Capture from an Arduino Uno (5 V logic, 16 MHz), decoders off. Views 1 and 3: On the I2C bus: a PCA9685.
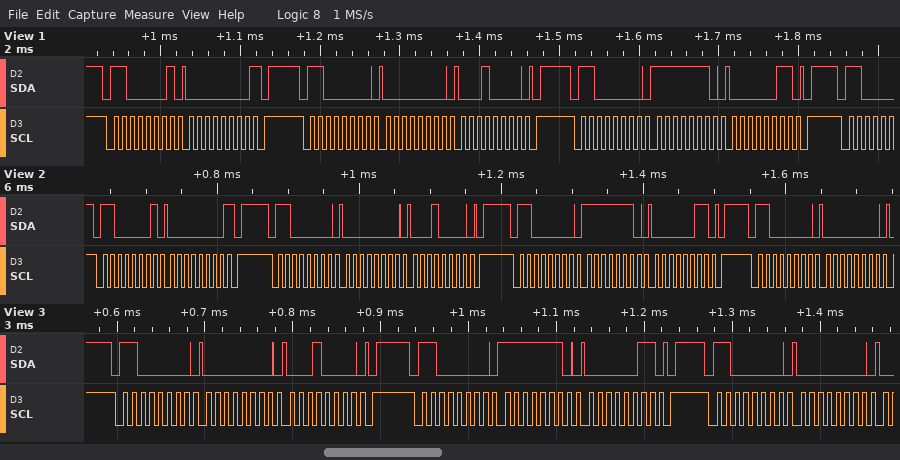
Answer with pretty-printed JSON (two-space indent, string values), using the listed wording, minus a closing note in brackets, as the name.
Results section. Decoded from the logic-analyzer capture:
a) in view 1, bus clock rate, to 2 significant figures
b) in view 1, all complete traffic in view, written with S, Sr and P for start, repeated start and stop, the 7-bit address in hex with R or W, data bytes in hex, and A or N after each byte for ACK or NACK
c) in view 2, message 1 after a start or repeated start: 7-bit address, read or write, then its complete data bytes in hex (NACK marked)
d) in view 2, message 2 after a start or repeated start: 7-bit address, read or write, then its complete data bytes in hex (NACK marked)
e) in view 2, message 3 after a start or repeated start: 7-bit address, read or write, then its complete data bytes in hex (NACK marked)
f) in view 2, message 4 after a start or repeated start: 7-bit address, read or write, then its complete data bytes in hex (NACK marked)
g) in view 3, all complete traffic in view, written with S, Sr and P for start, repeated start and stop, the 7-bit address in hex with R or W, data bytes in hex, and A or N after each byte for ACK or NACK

{
  "in view 1, bus clock rate, to 2 significant figures": "100 kHz",
  "in view 1, all complete traffic in view, written with S, Sr and P for start, repeated start and stop, the 7-bit address in hex with R or W, data bytes in hex, and A or N after each byte for ACK or NACK": "S 60R A 00 N P S 60W A 00 A 10 A P S 60W A FE A 03 A P",
  "in view 2, message 1 after a start or repeated start: 7-bit address, read or write, then its complete data bytes in hex": "0x60 read: 00 NACK",
  "in view 2, message 2 after a start or repeated start: 7-bit address, read or write, then its complete data bytes in hex": "0x60 write: 00 10",
  "in view 2, message 3 after a start or repeated start: 7-bit address, read or write, then its complete data bytes in hex": "0x60 write: FE 03",
  "in view 2, message 4 after a start or repeated start: 7-bit address, read or write, then its complete data bytes in hex": "0x60 write: 00",
  "in view 3, all complete traffic in view, written with S, Sr and P for start, repeated start and stop, the 7-bit address in hex with R or W, data bytes in hex, and A or N after each byte for ACK or NACK": "S 60W A 00 A 10 A P S 60W A FE A 03 A P S 60W A 00 A"
}
